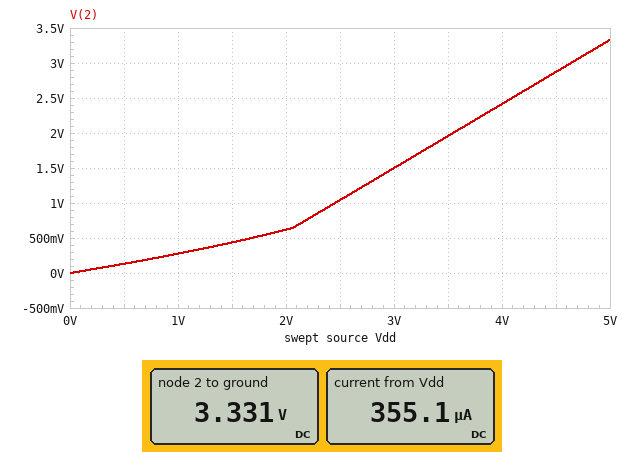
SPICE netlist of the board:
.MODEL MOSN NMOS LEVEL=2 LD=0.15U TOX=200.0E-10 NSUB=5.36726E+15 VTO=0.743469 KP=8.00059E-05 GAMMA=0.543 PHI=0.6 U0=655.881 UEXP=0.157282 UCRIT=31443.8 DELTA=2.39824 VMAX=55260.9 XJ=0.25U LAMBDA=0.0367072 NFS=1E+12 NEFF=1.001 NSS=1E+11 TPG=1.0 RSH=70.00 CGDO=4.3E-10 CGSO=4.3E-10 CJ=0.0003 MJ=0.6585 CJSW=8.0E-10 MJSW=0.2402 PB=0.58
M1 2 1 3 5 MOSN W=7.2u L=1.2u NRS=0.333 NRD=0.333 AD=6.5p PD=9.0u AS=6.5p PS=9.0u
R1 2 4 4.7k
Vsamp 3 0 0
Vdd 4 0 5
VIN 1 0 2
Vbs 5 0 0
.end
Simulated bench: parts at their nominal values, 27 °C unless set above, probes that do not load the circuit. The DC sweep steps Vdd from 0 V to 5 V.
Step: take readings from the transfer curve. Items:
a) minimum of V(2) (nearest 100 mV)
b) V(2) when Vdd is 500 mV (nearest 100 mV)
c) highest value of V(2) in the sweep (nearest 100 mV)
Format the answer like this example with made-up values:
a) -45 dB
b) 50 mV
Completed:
a) 0 V
b) 100 mV
c) 3.3 V
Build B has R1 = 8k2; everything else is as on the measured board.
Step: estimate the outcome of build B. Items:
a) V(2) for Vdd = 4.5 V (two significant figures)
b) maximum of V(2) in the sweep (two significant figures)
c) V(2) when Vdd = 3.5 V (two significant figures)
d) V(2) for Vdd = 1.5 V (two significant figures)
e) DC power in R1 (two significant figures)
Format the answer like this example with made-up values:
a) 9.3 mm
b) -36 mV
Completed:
a) 1.8 V
b) 2.3 V
c) 970 mV
d) 270 mV
e) 920 µW
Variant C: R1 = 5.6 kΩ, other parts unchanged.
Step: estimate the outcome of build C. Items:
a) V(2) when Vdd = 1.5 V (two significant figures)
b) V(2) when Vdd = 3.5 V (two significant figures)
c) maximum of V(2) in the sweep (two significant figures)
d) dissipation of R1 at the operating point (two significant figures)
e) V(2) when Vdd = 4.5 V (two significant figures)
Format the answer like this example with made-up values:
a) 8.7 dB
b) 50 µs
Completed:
a) 380 mV
b) 1.7 V
c) 3.0 V
d) 680 µW
e) 2.6 V
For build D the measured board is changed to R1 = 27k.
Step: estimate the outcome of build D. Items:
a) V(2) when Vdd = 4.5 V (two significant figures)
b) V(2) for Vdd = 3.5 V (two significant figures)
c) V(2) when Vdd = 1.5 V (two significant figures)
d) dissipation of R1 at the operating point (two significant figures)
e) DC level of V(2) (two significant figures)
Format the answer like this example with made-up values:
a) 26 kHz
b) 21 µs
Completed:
a) 280 mV
b) 210 mV
c) 87 mV
d) 810 µW
e) 320 mV
